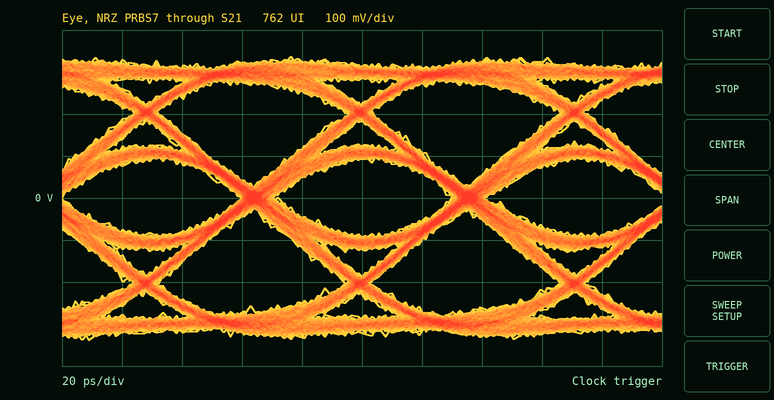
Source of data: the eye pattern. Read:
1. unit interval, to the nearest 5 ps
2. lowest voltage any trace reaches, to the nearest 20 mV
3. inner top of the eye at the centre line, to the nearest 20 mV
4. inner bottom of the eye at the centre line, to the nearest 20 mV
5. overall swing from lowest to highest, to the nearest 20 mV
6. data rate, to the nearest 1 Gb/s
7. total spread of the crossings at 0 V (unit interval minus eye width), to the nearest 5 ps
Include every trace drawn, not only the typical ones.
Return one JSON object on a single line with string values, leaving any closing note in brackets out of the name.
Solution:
{"unit interval, to the nearest 5 ps": "70 ps", "lowest voltage any trace reaches, to the nearest 20 mV": "-340 mV", "inner top of the eye at the centre line, to the nearest 20 mV": "100 mV", "inner bottom of the eye at the centre line, to the nearest 20 mV": "-100 mV", "overall swing from lowest to highest, to the nearest 20 mV": "680 mV", "data rate, to the nearest 1 Gb/s": "14 Gb/s", "total spread of the crossings at 0 V (unit interval minus eye width), to the nearest 5 ps": "15 ps"}
